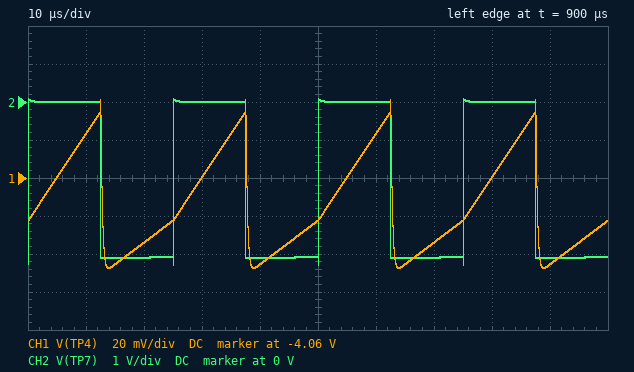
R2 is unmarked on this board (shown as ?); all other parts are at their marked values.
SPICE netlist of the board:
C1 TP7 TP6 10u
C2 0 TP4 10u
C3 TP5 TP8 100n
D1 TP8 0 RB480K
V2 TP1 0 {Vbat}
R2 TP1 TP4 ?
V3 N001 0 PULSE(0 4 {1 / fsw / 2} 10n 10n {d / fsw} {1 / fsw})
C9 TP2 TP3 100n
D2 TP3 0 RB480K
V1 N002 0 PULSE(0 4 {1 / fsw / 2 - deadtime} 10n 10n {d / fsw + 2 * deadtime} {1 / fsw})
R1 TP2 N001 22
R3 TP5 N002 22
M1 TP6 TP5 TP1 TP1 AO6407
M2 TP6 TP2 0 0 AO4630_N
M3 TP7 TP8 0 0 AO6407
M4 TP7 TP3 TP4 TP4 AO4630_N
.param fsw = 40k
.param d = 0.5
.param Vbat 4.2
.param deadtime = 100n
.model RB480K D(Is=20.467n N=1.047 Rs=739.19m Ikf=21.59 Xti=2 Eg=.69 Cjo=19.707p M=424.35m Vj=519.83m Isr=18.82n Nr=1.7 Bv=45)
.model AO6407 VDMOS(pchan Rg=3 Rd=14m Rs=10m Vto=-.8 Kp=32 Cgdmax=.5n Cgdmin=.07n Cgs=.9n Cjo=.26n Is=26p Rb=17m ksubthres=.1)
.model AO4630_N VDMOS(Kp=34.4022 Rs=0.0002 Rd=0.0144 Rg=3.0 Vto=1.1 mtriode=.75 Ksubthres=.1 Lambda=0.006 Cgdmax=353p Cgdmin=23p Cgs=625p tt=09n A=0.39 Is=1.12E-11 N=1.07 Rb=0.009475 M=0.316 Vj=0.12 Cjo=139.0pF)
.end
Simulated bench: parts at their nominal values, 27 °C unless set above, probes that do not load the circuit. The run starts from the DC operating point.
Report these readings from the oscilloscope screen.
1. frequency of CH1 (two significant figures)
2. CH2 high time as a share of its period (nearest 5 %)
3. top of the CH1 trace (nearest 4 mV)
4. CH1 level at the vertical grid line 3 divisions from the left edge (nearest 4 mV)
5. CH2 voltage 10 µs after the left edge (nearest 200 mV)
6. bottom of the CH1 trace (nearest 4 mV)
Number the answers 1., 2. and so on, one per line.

1. 40 kHz
2. 50 %
3. -4.020 V
4. -4.060 V
5. 0 V
6. -4.108 V
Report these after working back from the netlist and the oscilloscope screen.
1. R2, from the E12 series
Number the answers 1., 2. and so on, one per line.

1. 180 Ω
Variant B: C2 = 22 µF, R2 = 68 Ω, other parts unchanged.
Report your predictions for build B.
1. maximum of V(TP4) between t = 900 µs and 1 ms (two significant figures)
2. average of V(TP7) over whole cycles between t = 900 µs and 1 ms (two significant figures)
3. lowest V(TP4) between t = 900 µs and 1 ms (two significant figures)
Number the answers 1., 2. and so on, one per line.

1. -3.8 V
2. -2.0 V
3. -3.9 V
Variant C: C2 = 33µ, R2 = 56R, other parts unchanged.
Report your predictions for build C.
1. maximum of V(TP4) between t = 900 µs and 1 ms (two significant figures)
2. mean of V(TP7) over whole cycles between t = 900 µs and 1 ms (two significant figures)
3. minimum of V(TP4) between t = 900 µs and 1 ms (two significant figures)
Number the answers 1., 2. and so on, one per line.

1. -3.8 V
2. -1.9 V
3. -3.9 V
